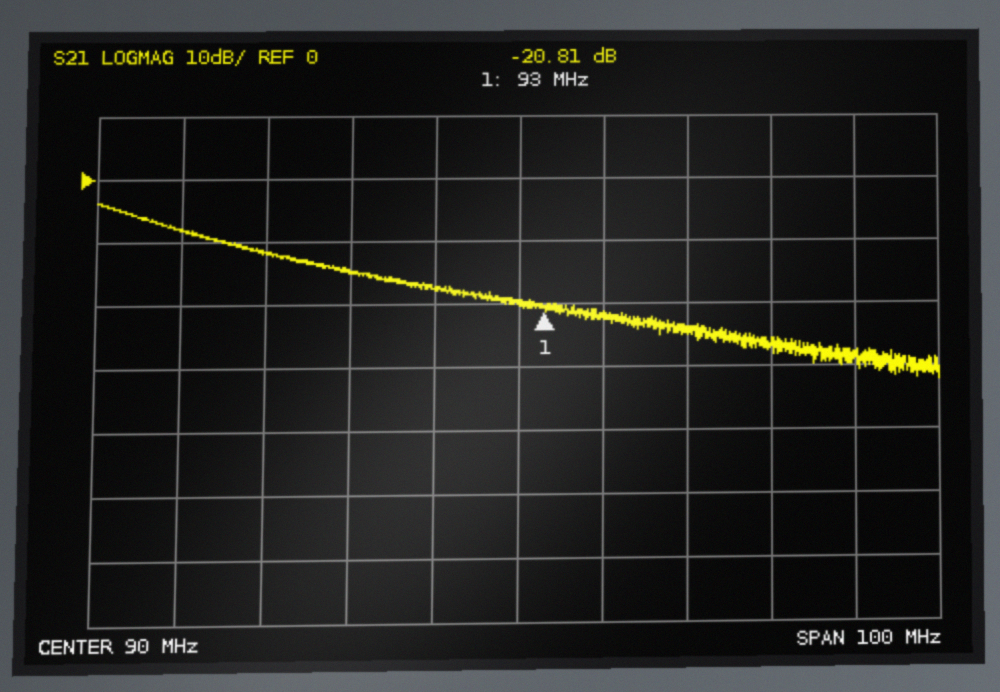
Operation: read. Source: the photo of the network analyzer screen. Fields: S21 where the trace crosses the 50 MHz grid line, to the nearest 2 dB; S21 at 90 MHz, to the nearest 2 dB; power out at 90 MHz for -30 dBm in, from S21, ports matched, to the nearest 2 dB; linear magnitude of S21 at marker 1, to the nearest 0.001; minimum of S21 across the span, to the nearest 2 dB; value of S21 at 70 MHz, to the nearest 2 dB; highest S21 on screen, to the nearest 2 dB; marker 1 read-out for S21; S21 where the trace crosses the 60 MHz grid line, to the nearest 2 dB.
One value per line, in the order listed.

-8 dB
-20 dB
-50 dBm
0.091
-32 dB
-14 dB
-4 dB
-20.81 dB
-12 dB
